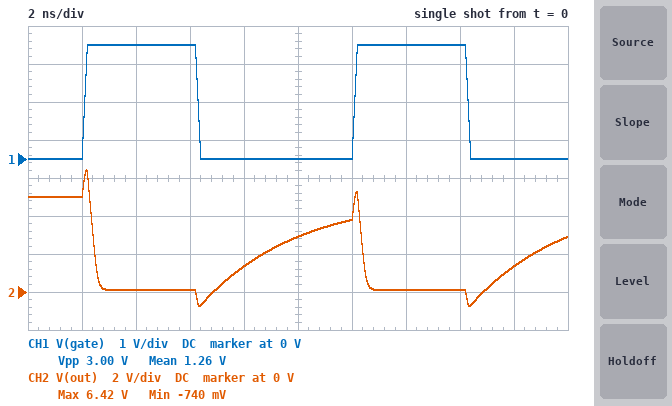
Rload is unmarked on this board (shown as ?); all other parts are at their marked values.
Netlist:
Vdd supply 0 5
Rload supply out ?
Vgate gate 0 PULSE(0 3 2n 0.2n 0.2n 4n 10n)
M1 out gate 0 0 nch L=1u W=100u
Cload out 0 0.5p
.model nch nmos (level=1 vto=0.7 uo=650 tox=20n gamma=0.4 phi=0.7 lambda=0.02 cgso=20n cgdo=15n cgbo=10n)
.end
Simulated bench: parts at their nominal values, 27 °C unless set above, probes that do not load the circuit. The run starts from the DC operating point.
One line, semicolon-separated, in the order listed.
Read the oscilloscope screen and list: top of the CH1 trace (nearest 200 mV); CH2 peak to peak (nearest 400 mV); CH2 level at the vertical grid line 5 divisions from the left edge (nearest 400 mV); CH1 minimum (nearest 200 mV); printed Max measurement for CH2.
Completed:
3.0 V; 7.2 V; 2.8 V; 0 V; 6.42 V
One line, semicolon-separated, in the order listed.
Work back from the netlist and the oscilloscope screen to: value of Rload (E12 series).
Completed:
1.8 kΩ
